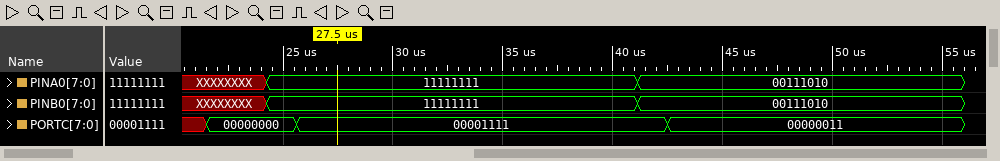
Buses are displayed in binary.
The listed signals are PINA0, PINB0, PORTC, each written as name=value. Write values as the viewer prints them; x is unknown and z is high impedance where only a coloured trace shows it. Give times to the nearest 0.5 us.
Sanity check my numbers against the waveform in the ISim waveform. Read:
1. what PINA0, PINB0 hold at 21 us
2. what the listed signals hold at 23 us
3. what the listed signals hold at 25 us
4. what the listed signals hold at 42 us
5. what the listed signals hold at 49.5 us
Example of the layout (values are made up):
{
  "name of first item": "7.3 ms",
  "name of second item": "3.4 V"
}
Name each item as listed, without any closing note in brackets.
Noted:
{
  "what PINA0, PINB0 hold at 21 us": "PINA0=XXXXXXXX, PINB0=XXXXXXXX",
  "what the listed signals hold at 23 us": "PINA0=XXXXXXXX, PINB0=XXXXXXXX, PORTC=00000000",
  "what the listed signals hold at 25 us": "PINA0=11111111, PINB0=11111111, PORTC=00000000",
  "what the listed signals hold at 42 us": "PINA0=00111010, PINB0=00111010, PORTC=00001111",
  "what the listed signals hold at 49.5 us": "PINA0=00111010, PINB0=00111010, PORTC=00000011"
}
